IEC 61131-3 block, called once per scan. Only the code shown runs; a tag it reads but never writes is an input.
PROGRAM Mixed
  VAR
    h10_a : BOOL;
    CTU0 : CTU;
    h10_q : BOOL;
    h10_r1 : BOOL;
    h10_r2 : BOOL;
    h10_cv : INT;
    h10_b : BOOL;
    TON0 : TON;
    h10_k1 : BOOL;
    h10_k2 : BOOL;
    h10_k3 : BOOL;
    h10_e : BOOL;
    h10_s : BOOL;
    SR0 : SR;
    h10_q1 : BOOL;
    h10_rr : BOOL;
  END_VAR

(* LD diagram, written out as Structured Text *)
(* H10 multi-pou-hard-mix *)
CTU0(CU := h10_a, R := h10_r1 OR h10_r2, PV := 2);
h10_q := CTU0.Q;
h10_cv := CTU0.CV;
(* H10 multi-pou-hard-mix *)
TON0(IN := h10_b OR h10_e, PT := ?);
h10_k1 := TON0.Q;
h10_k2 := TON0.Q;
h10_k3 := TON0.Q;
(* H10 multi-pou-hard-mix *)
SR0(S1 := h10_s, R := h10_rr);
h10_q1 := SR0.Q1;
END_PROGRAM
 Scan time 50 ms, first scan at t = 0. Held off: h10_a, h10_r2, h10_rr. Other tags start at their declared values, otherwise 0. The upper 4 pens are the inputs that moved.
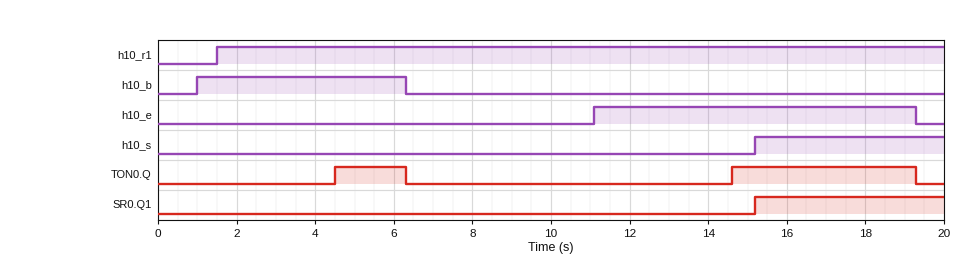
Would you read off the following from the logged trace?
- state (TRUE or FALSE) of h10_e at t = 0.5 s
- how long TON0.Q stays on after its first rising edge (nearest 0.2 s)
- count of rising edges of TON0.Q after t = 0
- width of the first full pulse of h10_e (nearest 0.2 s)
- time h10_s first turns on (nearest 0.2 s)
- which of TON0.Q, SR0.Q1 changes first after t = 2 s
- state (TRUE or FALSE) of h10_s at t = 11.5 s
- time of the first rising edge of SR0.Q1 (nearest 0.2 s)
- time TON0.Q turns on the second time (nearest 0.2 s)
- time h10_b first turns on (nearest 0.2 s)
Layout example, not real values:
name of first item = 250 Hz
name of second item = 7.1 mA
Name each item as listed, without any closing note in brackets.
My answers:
state (TRUE or FALSE) of h10_e at t = 0.5 s = FALSE
how long TON0.Q stays on after its first rising edge = 1.8 s
count of rising edges of TON0.Q after t = 0 = 2
width of the first full pulse of h10_e = 8.2 s
time h10_s first turns on = 15.2 s
which of TON0.Q, SR0.Q1 changes first after t = 2 s = TON0.Q
state (TRUE or FALSE) of h10_s at t = 11.5 s = FALSE
time of the first rising edge of SR0.Q1 = 15.2 s
time TON0.Q turns on the second time = 14.6 s
time h10_b first turns on = 1.0 s
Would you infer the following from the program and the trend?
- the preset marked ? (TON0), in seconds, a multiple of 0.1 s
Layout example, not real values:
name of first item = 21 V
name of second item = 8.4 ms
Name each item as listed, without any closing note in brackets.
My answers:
the preset marked ? (TON0), in seconds, a multiple of 0.1 s = 3.5 s
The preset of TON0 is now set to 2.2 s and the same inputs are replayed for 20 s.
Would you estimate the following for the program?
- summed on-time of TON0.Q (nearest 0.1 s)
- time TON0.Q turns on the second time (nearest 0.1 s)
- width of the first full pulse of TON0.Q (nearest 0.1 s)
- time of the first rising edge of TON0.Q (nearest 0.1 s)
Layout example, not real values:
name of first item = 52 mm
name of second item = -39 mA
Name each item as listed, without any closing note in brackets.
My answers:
summed on-time of TON0.Q = 9.1 s
time TON0.Q turns on the second time = 13.3 s
width of the first full pulse of TON0.Q = 3.1 s
time of the first rising edge of TON0.Q = 3.2 s
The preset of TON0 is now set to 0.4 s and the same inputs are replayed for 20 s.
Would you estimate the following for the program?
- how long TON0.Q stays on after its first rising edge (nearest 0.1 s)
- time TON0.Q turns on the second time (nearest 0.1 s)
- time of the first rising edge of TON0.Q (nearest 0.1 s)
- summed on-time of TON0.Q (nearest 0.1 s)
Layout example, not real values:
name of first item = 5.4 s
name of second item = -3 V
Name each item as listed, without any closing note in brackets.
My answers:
how long TON0.Q stays on after its first rising edge = 4.9 s
time TON0.Q turns on the second time = 11.5 s
time of the first rising edge of TON0.Q = 1.4 s
summed on-time of TON0.Q = 12.7 s
